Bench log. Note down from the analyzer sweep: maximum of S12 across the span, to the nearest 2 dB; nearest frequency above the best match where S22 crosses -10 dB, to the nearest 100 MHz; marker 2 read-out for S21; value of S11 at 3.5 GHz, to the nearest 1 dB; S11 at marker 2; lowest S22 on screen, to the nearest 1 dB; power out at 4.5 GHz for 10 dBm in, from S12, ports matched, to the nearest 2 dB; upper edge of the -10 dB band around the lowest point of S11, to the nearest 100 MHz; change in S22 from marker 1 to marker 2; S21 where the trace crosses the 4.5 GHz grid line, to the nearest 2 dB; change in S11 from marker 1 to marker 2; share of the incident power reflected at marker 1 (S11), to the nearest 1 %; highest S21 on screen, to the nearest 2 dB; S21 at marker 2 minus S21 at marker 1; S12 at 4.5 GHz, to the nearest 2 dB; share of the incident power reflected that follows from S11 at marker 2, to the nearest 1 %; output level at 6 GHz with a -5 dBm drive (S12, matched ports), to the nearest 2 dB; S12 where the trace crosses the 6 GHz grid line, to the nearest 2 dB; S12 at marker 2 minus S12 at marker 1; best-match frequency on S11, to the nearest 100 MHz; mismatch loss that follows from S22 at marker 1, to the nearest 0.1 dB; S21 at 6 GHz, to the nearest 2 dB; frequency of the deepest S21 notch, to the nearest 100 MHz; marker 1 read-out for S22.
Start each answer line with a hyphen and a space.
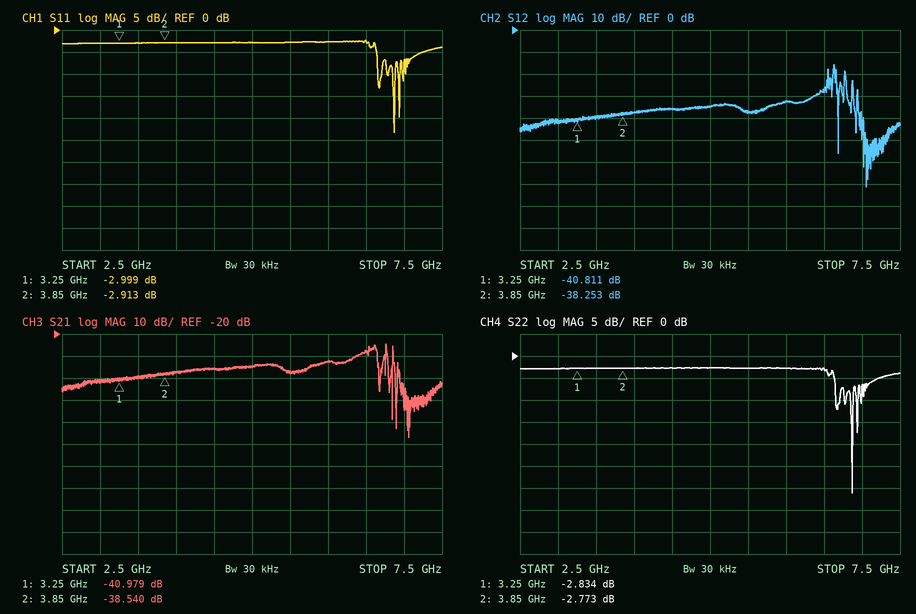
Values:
- -16 dB
- 6.9 GHz
- -38.540 dB
- -3 dB
- -2.913 dB
- -31 dB
- -26 dBm
- 6.9 GHz
- 0.061 dB
- -36 dB
- 0.086 dB
- 50 %
- -24 dB
- 2.439 dB
- -36 dB
- 51 %
- -38 dBm
- -32 dB
- 2.558 dB
- 6.9 GHz
- 3.2 dB
- -32 dB
- 7.1 GHz
- -2.834 dB
